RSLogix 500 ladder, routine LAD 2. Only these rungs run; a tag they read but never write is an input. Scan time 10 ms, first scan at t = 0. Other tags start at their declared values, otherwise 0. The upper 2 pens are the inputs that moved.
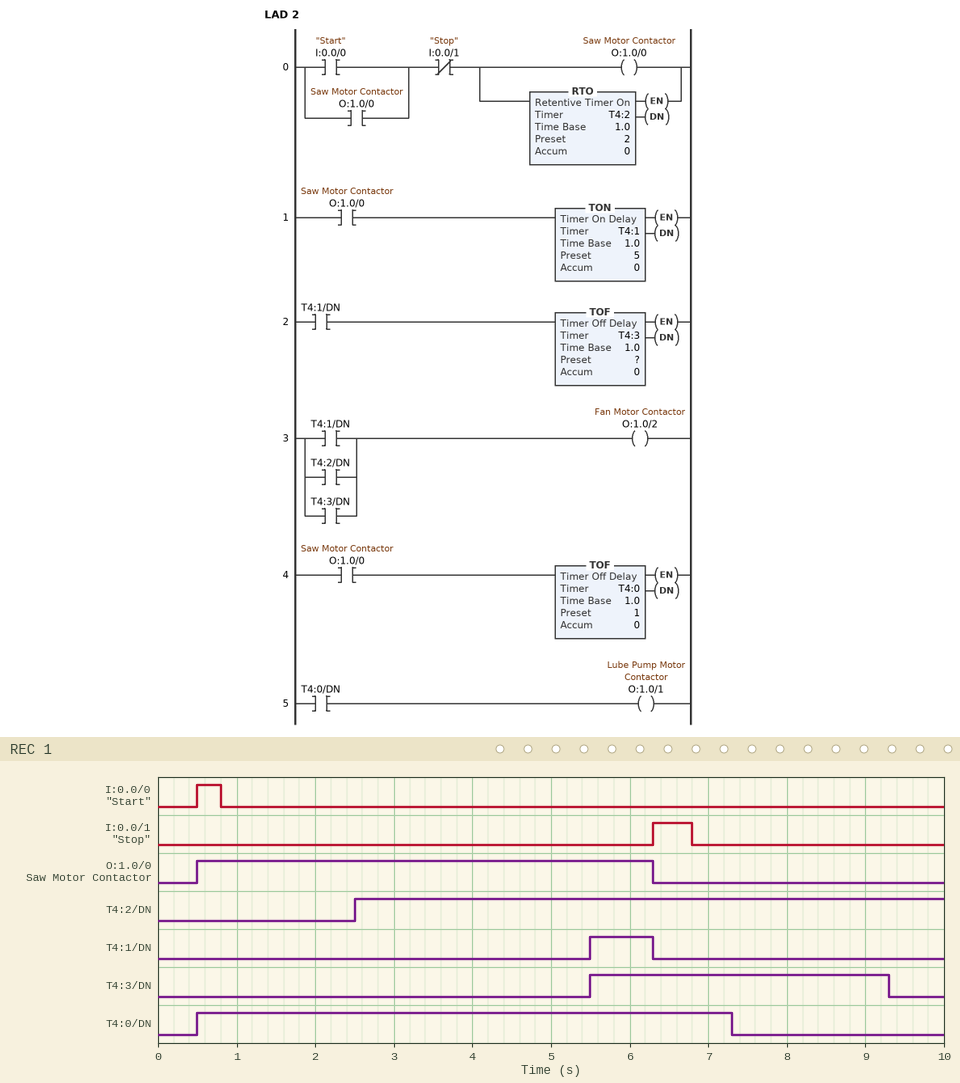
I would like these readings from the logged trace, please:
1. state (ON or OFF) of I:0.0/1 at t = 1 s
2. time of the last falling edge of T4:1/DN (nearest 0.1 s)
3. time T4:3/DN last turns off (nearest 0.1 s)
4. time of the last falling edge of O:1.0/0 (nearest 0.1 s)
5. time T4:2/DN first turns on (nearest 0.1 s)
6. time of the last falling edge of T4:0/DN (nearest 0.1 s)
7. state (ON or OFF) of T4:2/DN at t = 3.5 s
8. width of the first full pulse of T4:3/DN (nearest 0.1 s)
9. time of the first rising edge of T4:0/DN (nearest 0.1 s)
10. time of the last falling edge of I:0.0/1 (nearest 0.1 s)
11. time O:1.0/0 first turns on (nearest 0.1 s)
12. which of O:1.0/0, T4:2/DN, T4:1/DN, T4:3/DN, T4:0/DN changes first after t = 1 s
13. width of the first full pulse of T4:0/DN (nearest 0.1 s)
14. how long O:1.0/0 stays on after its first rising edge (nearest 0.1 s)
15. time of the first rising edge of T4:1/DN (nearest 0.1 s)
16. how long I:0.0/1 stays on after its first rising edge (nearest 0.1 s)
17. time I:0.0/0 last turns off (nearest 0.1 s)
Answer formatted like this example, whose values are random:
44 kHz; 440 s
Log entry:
OFF; 6.3 s; 9.3 s; 6.3 s; 2.5 s; 7.3 s; ON; 3.8 s; 0.5 s; 6.8 s; 0.5 s; T4:2/DN; 6.8 s; 5.8 s; 5.5 s; 0.5 s; 0.8 s
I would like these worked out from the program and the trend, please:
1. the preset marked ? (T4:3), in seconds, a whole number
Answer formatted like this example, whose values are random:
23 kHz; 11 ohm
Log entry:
3 s
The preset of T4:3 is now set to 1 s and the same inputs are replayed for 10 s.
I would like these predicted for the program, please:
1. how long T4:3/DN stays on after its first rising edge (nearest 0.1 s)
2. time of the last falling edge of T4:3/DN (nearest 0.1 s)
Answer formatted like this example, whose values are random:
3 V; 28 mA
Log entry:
1.8 s; 7.3 s
